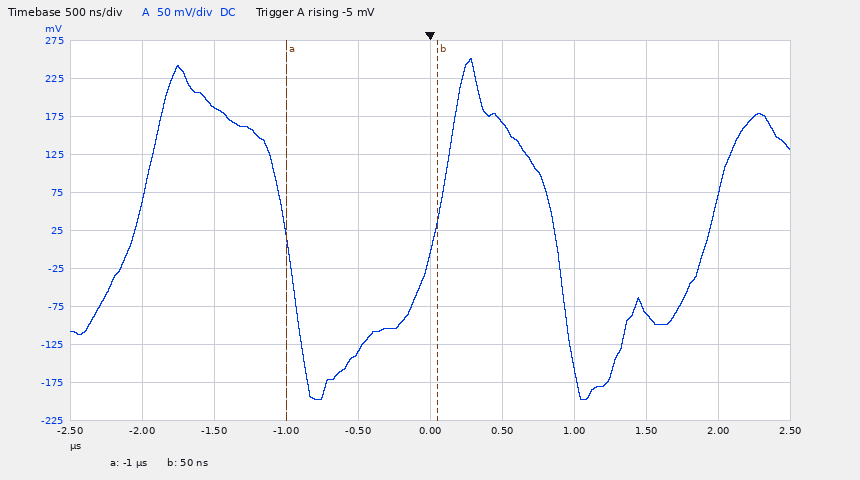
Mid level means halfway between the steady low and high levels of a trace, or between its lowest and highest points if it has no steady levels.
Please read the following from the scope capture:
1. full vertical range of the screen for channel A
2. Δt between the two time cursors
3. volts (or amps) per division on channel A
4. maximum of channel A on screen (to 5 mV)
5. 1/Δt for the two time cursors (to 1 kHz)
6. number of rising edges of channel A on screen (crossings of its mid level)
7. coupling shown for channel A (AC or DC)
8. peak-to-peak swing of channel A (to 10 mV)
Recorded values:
500 mV
1.05 µs
50 mV
250 mV
952 kHz
3
DC
450 mV
